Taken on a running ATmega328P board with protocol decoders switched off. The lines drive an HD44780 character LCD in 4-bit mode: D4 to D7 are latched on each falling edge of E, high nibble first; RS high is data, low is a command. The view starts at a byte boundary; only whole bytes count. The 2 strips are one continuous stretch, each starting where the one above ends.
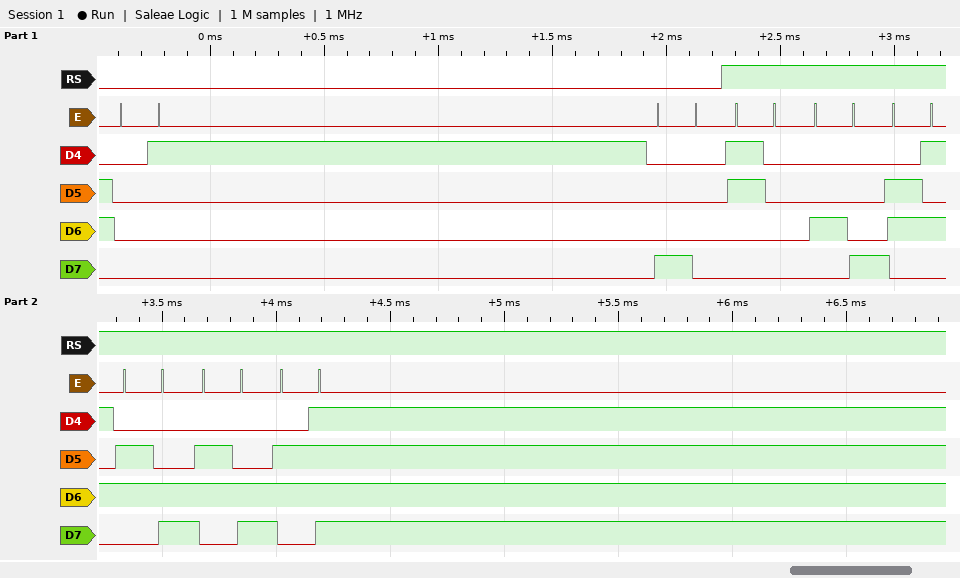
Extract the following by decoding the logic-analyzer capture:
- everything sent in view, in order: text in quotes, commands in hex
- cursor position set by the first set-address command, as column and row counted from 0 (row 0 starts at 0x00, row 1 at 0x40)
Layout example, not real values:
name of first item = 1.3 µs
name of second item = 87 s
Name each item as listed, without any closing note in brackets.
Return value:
everything sent in view, in order: text in quotes, commands in hex = 0x01 0x80 "0Hello"
cursor position set by the first set-address command, as column and row counted from 0 = column 0, row 0
